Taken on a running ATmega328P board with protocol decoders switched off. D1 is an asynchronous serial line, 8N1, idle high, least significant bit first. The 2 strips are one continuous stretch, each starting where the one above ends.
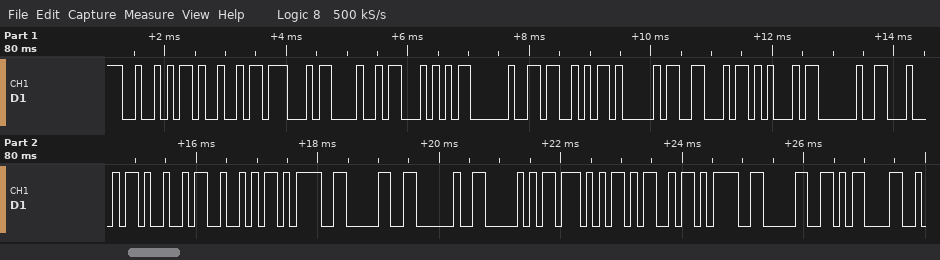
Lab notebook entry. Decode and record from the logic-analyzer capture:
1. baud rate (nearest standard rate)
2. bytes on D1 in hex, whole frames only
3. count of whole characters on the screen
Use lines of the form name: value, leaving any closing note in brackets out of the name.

baud rate: 9600 baud
bytes on D1 in hex, whole frames only: 52 49 47 48 54 20 53 41 46 45 20 44 49 52 3D 30 20 50 57 4D 3D 30 0D
count of whole characters on the screen: 23
